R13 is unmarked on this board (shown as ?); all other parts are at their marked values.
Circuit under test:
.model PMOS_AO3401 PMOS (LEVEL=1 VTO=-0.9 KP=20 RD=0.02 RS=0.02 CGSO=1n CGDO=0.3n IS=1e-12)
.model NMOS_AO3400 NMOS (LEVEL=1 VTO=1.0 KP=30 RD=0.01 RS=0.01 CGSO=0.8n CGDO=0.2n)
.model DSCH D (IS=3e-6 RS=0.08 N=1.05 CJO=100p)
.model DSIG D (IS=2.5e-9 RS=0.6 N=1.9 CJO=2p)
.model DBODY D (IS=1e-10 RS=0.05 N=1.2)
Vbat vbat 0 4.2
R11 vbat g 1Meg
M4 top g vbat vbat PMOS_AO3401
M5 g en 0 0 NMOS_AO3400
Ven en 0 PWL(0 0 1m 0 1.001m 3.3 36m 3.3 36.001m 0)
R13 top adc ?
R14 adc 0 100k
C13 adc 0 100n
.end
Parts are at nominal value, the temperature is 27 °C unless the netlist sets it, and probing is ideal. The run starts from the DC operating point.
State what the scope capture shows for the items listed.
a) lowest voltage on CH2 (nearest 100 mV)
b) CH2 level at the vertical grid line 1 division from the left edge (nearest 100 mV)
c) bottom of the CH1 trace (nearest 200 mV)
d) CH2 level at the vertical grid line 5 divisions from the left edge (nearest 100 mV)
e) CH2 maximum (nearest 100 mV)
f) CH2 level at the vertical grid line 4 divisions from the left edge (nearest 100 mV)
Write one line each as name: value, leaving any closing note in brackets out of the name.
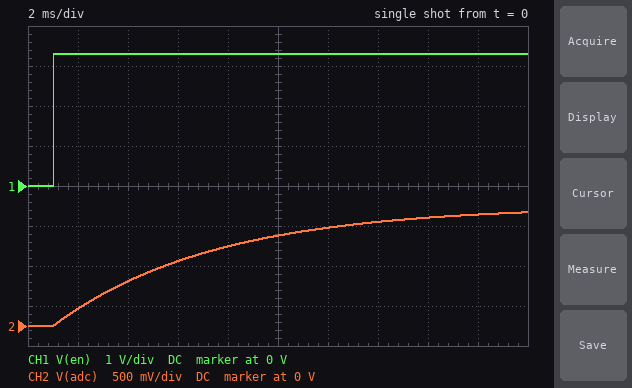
lowest voltage on CH2: 0 V
CH2 level at the vertical grid line 1 division from the left edge: 200 mV
bottom of the CH1 trace: 0 V
CH2 level at the vertical grid line 5 divisions from the left edge: 1.1 V
CH2 maximum: 1.4 V
CH2 level at the vertical grid line 4 divisions from the left edge: 1.0 V
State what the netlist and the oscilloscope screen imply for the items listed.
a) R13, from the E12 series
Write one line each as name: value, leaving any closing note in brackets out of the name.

R13, from the E12 series: 180 kΩ
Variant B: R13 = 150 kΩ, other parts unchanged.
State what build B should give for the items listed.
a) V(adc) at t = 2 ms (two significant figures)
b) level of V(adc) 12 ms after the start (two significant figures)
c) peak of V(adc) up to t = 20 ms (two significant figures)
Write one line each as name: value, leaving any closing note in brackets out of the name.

V(adc) at t = 2 ms: 260 mV
level of V(adc) 12 ms after the start: 1.4 V
peak of V(adc) up to t = 20 ms: 1.6 V
